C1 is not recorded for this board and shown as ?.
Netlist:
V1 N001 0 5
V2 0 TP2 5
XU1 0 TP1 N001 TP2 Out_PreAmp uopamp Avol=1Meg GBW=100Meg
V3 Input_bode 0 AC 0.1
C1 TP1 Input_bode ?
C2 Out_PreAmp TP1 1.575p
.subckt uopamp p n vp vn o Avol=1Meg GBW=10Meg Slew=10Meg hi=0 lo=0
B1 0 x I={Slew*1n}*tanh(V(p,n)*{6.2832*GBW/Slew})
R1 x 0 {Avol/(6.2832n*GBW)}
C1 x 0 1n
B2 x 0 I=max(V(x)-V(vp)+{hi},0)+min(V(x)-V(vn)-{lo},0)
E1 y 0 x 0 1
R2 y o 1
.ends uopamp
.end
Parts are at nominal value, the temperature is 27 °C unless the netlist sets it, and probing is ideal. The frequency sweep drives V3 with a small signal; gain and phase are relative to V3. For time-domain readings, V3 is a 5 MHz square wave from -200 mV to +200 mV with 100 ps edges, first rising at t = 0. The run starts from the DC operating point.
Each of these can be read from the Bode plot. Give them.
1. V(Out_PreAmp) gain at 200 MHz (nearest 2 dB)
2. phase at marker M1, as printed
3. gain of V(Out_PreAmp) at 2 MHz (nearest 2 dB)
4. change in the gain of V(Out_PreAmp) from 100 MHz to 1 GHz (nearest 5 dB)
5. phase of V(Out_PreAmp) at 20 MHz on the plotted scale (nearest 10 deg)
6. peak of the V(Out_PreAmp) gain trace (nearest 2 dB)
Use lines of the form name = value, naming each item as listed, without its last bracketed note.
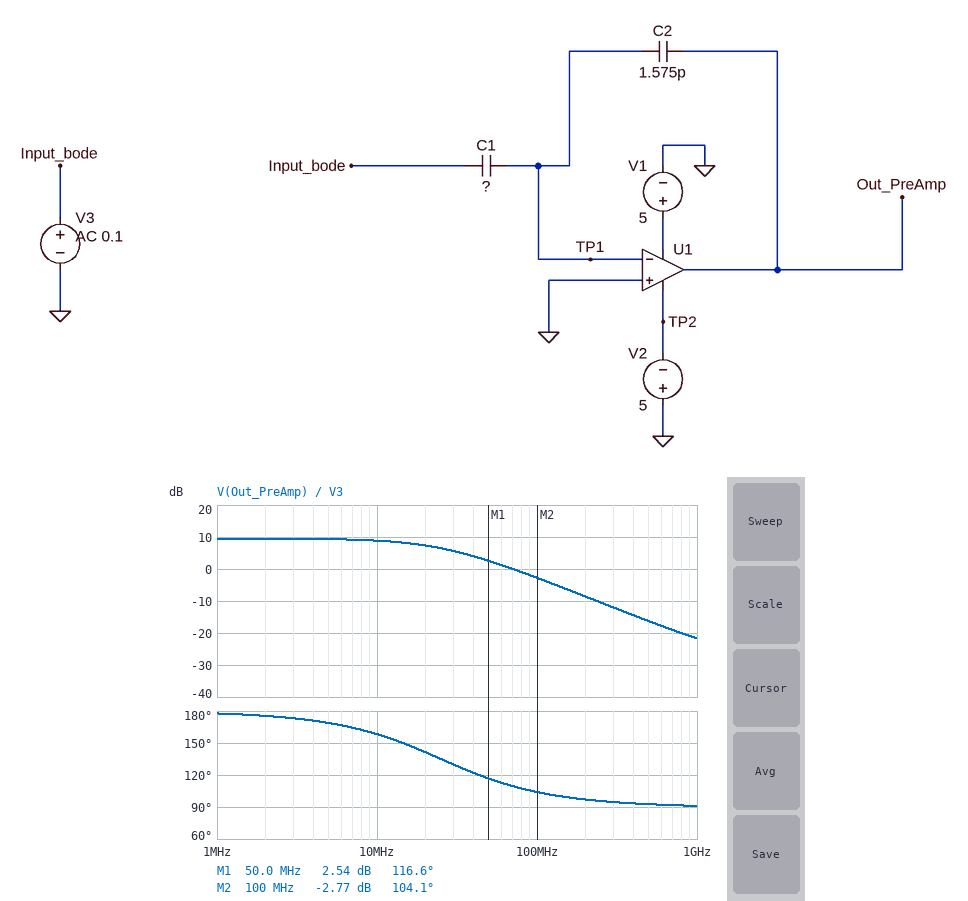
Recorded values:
V(Out_PreAmp) gain at 200 MHz = -8 dB
phase at marker M1, as printed = 116.6 deg
gain of V(Out_PreAmp) at 2 MHz = 10 dB
change in the gain of V(Out_PreAmp) from 100 MHz to 1 GHz = -20 dB
phase of V(Out_PreAmp) at 20 MHz on the plotted scale = 140 deg
peak of the V(Out_PreAmp) gain trace = 10 dB
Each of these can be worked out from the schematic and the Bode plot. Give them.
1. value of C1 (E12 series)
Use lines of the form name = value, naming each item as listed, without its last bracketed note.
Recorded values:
value of C1 = 4.7 pF
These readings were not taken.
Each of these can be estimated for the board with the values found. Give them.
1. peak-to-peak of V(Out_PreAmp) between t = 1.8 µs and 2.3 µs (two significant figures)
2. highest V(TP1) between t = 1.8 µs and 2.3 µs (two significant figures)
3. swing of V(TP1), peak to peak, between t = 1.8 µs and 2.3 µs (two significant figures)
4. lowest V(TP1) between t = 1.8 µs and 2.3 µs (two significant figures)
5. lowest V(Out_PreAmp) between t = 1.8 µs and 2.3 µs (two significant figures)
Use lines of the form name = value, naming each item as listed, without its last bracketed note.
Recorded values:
peak-to-peak of V(Out_PreAmp) between t = 1.8 µs and 2.3 µs = 1.0 V
highest V(TP1) between t = 1.8 µs and 2.3 µs = 280 mV
swing of V(TP1), peak to peak, between t = 1.8 µs and 2.3 µs = 550 mV
lowest V(TP1) between t = 1.8 µs and 2.3 µs = -270 mV
lowest V(Out_PreAmp) between t = 1.8 µs and 2.3 µs = -1.1 V
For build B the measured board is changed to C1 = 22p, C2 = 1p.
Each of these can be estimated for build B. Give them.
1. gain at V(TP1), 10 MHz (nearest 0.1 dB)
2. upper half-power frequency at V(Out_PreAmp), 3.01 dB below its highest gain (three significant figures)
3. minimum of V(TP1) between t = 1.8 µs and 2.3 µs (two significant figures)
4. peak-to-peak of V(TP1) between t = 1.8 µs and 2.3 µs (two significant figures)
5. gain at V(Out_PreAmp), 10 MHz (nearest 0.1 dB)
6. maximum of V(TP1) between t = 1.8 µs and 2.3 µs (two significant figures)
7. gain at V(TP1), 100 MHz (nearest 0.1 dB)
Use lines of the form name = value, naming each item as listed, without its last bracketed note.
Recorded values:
gain at V(TP1), 10 MHz = -1.1 dB
upper half-power frequency at V(Out_PreAmp), 3.01 dB below its highest gain = 4.35 MHz
minimum of V(TP1) between t = 1.8 µs and 2.3 µs = -68 mV
peak-to-peak of V(TP1) between t = 1.8 µs and 2.3 µs = 430 mV
gain at V(Out_PreAmp), 10 MHz = 18.9 dB
maximum of V(TP1) between t = 1.8 µs and 2.3 µs = 360 mV
gain at V(TP1), 100 MHz = -0.4 dB
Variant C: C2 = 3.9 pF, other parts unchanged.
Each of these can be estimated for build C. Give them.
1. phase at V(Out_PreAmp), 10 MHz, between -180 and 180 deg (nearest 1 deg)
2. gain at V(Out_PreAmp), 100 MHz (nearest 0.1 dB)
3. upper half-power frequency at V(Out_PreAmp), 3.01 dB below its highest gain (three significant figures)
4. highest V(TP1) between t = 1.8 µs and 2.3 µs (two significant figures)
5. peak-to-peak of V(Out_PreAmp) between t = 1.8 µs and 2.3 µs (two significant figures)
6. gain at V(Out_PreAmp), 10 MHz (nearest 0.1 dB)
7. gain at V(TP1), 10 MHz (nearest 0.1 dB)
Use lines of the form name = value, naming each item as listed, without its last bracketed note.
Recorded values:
phase at V(Out_PreAmp), 10 MHz, between -180 and 180 deg = 168 deg
gain at V(Out_PreAmp), 100 MHz = -6.0 dB
upper half-power frequency at V(Out_PreAmp), 3.01 dB below its highest gain = 45.4 MHz
highest V(TP1) between t = 1.8 µs and 2.3 µs = 220 mV
peak-to-peak of V(Out_PreAmp) between t = 1.8 µs and 2.3 µs = 500 mV
gain at V(Out_PreAmp), 10 MHz = 1.4 dB
gain at V(TP1), 10 MHz = -18.6 dB
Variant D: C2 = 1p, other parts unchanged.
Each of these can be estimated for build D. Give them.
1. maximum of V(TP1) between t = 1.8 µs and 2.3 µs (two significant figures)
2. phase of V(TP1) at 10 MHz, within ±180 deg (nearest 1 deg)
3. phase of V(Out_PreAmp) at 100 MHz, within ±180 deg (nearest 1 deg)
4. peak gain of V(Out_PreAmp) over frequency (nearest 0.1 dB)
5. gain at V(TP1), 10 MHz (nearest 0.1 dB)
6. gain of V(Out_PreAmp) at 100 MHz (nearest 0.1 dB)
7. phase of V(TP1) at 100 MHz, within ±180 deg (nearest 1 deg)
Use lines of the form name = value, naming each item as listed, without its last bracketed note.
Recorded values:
maximum of V(TP1) between t = 1.8 µs and 2.3 µs = 310 mV
phase of V(TP1) at 10 MHz, within ±180 deg = 60 deg
phase of V(Out_PreAmp) at 100 MHz, within ±180 deg = 100 deg
peak gain of V(Out_PreAmp) over frequency = 13.4 dB
gain at V(TP1), 10 MHz = -7.8 dB
gain of V(Out_PreAmp) at 100 MHz = -1.8 dB
phase of V(TP1) at 100 MHz, within ±180 deg = 10 deg
